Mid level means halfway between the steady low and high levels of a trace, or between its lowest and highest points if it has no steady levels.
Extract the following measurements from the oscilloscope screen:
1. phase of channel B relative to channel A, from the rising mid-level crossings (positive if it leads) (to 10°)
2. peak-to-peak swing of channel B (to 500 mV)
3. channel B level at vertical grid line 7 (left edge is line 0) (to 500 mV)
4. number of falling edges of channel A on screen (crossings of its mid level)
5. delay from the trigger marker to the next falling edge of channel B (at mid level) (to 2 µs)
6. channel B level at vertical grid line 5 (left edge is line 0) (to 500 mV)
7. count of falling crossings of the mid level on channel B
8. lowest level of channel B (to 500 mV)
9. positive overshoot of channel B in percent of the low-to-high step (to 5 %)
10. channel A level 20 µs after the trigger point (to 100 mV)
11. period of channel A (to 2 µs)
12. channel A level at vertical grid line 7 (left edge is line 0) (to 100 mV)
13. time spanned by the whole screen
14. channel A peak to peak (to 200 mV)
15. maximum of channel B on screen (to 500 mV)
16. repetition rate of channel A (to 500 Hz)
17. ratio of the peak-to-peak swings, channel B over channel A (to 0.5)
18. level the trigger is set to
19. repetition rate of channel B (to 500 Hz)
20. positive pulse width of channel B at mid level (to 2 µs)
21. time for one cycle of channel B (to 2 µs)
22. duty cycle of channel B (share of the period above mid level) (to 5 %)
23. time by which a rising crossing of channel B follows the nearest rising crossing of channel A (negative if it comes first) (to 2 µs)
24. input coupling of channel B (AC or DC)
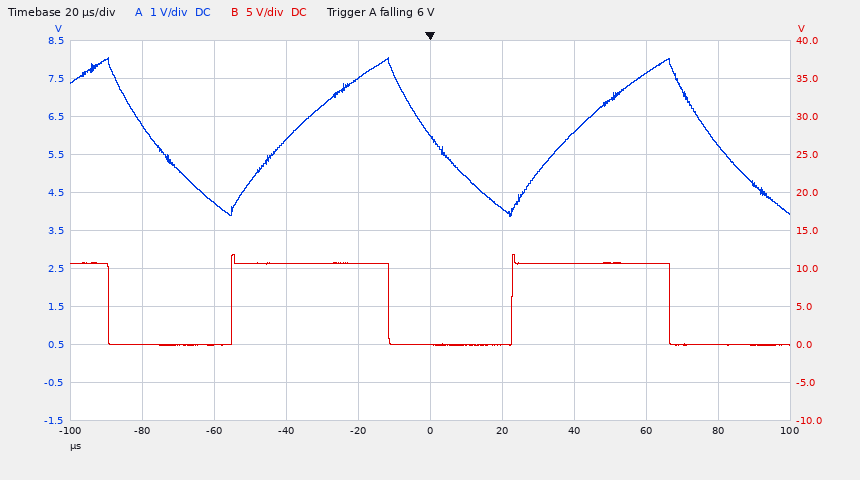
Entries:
+70°
12.0 V
10.5 V
3
66 µs
0.0 V
3
0.0 V
10 %
4.1 V
78 µs
6.1 V
200 µs
4.2 V
12.0 V
13.0 kHz
3.0
6 V
13.0 kHz
44 µs
78 µs
55 %
-16 µs
DC
